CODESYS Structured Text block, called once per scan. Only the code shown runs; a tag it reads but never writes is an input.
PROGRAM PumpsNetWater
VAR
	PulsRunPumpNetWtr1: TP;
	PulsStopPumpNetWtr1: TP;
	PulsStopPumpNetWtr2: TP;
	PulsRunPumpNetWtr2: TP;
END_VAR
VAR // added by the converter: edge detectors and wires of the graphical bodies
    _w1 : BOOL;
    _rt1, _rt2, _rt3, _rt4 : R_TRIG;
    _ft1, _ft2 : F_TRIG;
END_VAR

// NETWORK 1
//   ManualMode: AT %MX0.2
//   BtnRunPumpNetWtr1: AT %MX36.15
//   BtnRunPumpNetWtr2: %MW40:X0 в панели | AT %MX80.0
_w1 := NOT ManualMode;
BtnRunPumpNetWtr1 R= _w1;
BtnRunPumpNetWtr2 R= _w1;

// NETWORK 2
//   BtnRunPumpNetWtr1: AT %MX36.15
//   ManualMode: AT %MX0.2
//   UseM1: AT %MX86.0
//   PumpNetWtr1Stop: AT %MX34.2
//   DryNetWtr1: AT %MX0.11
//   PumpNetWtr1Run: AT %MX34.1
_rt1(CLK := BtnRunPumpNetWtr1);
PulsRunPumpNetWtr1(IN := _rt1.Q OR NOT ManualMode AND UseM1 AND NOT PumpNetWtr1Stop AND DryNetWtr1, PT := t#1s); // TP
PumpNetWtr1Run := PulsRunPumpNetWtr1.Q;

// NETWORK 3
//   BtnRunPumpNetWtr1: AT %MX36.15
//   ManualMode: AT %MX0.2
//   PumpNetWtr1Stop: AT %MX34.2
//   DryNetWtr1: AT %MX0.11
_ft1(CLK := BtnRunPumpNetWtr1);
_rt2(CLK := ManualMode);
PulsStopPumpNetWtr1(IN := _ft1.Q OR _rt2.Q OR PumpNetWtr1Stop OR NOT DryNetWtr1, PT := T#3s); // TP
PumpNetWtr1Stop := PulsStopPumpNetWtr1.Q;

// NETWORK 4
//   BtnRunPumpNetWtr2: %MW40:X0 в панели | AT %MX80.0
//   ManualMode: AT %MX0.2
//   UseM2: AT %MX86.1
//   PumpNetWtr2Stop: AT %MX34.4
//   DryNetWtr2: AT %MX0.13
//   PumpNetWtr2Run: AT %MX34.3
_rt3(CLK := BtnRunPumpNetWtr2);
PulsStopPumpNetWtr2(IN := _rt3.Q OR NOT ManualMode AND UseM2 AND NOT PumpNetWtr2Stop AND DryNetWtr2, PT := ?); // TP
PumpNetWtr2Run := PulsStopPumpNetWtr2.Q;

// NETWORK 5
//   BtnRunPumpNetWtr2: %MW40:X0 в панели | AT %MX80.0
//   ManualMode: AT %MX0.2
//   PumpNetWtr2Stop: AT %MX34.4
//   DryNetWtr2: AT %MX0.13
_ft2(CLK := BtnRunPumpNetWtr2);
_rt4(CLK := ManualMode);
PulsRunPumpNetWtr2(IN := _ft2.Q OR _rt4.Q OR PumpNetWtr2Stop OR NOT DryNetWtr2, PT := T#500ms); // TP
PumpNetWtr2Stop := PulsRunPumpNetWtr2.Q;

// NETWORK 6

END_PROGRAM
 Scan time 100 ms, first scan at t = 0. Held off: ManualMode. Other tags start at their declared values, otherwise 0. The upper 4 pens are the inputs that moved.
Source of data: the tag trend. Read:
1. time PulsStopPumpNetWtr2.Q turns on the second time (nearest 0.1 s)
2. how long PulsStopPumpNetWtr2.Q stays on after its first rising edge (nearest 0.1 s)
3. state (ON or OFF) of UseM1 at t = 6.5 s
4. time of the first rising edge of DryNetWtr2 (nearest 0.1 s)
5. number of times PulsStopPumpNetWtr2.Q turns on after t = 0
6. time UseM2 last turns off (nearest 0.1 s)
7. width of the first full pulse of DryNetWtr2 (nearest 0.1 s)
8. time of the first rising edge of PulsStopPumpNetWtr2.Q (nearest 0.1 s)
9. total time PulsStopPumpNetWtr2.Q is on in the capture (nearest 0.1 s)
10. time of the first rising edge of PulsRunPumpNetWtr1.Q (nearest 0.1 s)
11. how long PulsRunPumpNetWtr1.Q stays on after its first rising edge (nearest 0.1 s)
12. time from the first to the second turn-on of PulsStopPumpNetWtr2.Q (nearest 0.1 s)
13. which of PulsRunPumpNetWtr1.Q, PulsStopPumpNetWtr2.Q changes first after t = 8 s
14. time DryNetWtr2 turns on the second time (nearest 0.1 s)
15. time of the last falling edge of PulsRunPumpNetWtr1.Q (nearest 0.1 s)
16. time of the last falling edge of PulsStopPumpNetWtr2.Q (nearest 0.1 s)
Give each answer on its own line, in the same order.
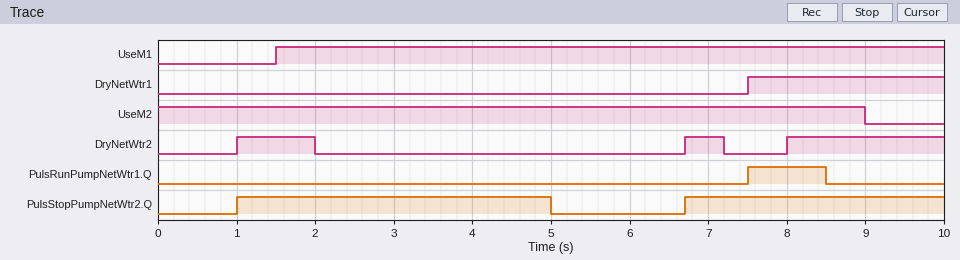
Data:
6.7 s
4.0 s
ON
1.0 s
2
9.0 s
1.0 s
1.0 s
7.3 s
7.5 s
1.0 s
5.7 s
PulsRunPumpNetWtr1.Q
6.7 s
8.5 s
5.0 s
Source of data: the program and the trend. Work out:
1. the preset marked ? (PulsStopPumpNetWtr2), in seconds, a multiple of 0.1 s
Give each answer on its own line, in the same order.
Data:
4.0 s
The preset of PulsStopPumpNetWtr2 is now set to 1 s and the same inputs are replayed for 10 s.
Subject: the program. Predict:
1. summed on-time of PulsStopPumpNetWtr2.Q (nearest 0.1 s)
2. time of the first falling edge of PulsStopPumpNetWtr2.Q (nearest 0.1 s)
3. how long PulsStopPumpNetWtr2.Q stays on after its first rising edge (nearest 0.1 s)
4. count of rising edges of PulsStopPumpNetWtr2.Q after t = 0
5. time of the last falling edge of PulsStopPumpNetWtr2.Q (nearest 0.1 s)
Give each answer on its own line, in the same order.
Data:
3.0 s
2.0 s
1.0 s
3
9.0 s
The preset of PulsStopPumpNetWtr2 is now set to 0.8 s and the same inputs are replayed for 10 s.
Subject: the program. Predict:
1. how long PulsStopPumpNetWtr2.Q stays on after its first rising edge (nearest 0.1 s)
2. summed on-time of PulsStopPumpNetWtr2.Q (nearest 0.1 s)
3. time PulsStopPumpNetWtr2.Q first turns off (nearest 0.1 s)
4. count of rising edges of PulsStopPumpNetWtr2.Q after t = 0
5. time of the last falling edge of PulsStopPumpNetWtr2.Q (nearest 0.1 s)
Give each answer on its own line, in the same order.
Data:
0.8 s
2.4 s
1.8 s
3
8.8 s
